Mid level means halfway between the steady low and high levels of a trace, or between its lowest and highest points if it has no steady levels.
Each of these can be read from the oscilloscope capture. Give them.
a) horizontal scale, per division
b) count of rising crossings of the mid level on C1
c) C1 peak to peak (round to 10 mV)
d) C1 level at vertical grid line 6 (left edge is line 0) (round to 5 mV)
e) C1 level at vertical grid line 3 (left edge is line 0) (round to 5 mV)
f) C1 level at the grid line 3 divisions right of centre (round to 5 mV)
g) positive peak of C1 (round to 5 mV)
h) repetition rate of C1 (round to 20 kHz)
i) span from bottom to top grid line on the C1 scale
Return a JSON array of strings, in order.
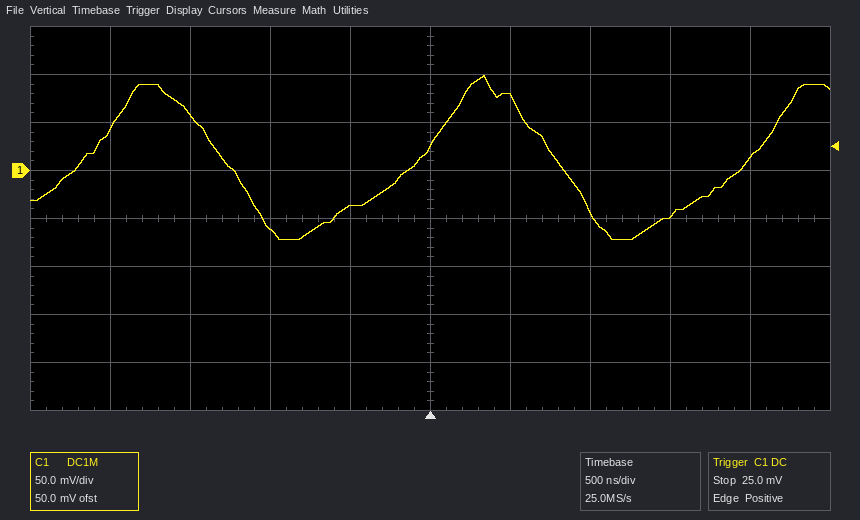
["500 ns", "3", "170 mV", "75 mV", "-60 mV", "-45 mV", "100 mV", "480 kHz", "400 mV"]
